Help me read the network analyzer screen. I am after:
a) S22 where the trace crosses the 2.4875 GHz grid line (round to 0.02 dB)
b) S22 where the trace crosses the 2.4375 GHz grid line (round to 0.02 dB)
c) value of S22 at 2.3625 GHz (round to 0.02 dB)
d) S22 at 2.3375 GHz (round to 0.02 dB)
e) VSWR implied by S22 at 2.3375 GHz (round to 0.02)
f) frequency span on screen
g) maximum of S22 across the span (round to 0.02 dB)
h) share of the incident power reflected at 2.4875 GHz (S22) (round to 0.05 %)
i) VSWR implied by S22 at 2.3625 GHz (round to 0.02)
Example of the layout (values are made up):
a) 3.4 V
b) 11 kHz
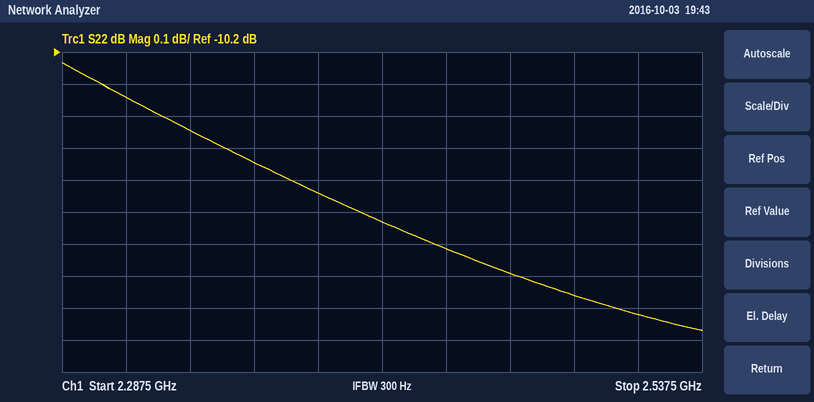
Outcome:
a) -10.96 dB
b) -10.82 dB
c) -10.54 dB
d) -10.44 dB
e) 1.86
f) 250 MHz
g) -10.24 dB
h) 8.00 %
i) 1.84
